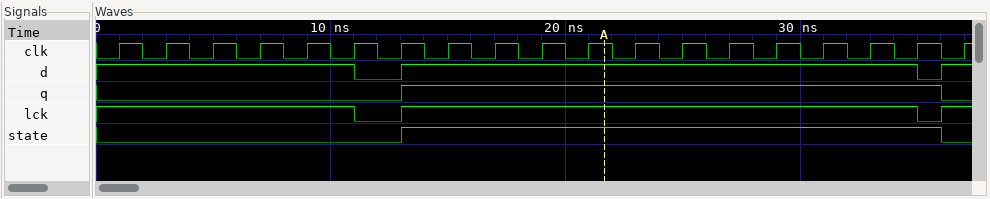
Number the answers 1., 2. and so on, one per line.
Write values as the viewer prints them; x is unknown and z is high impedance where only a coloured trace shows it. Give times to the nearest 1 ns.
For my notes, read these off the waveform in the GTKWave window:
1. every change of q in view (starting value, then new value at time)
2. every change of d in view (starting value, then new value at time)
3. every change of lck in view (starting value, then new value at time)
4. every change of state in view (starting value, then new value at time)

1. 0, 1 at 13 ns, 0 at 36 ns
2. 1, 0 at 11 ns, 1 at 13 ns, 0 at 35 ns, 1 at 36 ns
3. 1, 0 at 11 ns, 1 at 13 ns, 0 at 35 ns, 1 at 36 ns
4. 0, 1 at 13 ns, 0 at 36 ns
